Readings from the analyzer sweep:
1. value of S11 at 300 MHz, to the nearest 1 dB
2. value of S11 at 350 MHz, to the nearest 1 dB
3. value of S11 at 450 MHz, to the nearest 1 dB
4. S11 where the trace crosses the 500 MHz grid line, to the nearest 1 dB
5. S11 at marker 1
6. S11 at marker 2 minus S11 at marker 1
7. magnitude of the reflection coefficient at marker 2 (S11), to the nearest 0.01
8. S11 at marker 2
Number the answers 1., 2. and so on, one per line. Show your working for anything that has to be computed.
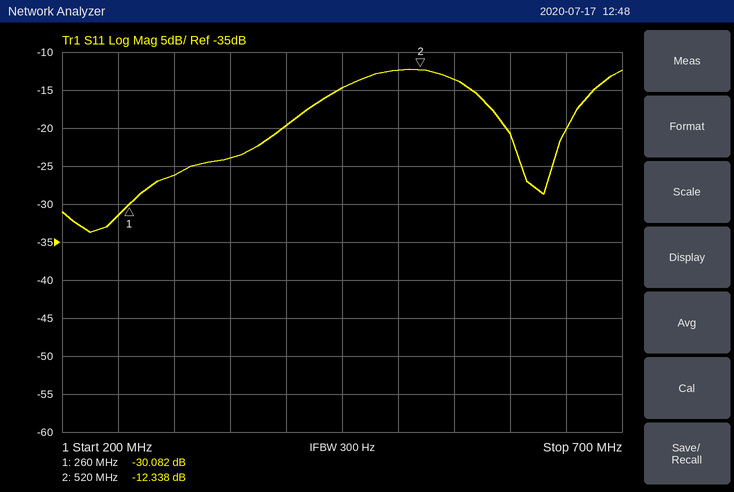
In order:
1. -26 dB
2. -24 dB
3. -15 dB
4. -12 dB
5. -30.082 dB
6. -12.338 − (-30.082) = 17.744 dB
7. 10^(-12.338/20) ≈ 0.24
8. -12.338 dB
